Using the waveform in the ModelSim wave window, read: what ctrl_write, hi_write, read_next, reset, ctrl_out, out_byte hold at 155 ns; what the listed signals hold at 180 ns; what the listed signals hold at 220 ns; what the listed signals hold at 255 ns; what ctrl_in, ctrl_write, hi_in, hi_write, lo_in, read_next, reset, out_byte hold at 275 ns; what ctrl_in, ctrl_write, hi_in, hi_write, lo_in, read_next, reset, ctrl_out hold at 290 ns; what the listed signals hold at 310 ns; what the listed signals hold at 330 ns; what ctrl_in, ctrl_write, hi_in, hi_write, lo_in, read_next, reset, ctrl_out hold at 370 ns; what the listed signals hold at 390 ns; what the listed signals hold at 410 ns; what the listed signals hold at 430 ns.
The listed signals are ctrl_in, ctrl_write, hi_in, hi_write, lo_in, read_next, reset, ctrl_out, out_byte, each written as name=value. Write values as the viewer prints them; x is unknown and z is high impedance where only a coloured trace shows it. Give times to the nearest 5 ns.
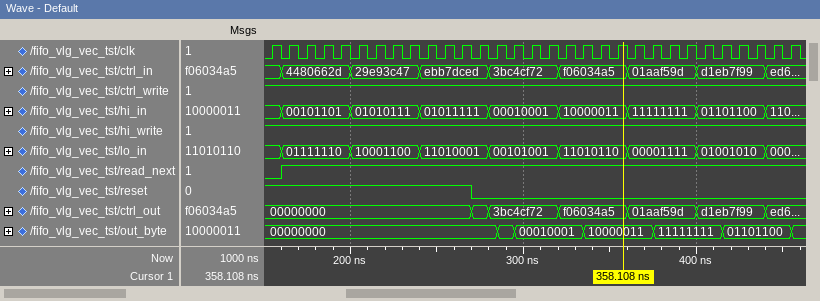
ctrl_write=1, hi_write=1, read_next=0, reset=1, ctrl_out=00000000, out_byte=00000000
ctrl_in=4480662d, ctrl_write=1, hi_in=00101101, hi_write=1, lo_in=01111110, read_next=1, reset=1, ctrl_out=00000000, out_byte=00000000
ctrl_in=29e93c47, ctrl_write=1, hi_in=01010111, hi_write=1, lo_in=10001100, read_next=1, reset=1, ctrl_out=00000000, out_byte=00000000
ctrl_in=ebb7dced, ctrl_write=1, hi_in=01011111, hi_write=1, lo_in=11010001, read_next=1, reset=1, ctrl_out=00000000, out_byte=00000000
ctrl_in=ebb7dced, ctrl_write=1, hi_in=01011111, hi_write=1, lo_in=11010001, read_next=1, reset=0, out_byte=00000000
ctrl_in=3bc4cf72, ctrl_write=1, hi_in=00010001, hi_write=1, lo_in=00101001, read_next=1, reset=0, ctrl_out=3bc4cf72
ctrl_in=3bc4cf72, ctrl_write=1, hi_in=00010001, hi_write=1, lo_in=00101001, read_next=1, reset=0, ctrl_out=3bc4cf72, out_byte=00010001
ctrl_in=f06034a5, ctrl_write=1, hi_in=10000011, hi_write=1, lo_in=11010110, read_next=1, reset=0, ctrl_out=f06034a5, out_byte=00010001
ctrl_in=01aaf59d, ctrl_write=1, hi_in=11111111, hi_write=1, lo_in=00001111, read_next=1, reset=0, ctrl_out=01aaf59d
ctrl_in=01aaf59d, ctrl_write=1, hi_in=11111111, hi_write=1, lo_in=00001111, read_next=1, reset=0, ctrl_out=01aaf59d, out_byte=11111111
ctrl_in=d1eb7f99, ctrl_write=1, hi_in=01101100, hi_write=1, lo_in=01001010, read_next=1, reset=0, ctrl_out=d1eb7f99, out_byte=11111111
ctrl_in=d1eb7f99, ctrl_write=1, hi_in=01101100, hi_write=1, lo_in=01001010, read_next=1, reset=0, ctrl_out=d1eb7f99, out_byte=01101100
